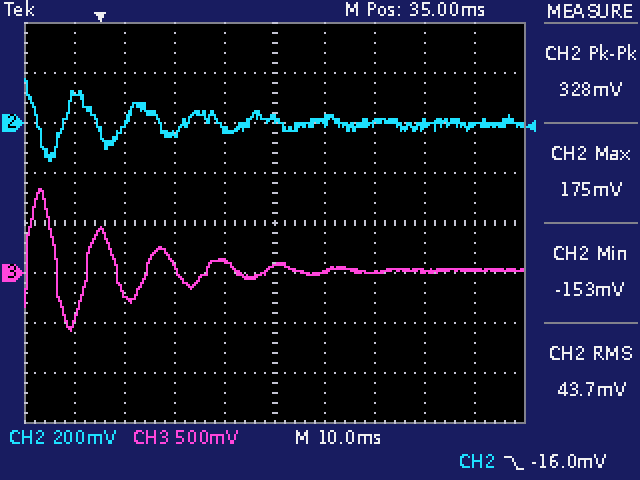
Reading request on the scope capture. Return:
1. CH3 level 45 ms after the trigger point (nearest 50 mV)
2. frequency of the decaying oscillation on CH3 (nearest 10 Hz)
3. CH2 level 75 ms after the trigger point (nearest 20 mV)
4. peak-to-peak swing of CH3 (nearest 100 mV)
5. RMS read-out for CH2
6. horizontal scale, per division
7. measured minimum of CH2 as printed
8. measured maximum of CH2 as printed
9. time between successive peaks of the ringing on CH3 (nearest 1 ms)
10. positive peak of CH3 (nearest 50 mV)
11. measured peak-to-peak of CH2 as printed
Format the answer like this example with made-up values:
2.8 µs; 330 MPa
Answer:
0 mV; 80 Hz; 0 mV; 1.40 V; 43.7 mV; 10 ms; -153 mV; 175 mV; 12 ms; 850 mV; 328 mV
